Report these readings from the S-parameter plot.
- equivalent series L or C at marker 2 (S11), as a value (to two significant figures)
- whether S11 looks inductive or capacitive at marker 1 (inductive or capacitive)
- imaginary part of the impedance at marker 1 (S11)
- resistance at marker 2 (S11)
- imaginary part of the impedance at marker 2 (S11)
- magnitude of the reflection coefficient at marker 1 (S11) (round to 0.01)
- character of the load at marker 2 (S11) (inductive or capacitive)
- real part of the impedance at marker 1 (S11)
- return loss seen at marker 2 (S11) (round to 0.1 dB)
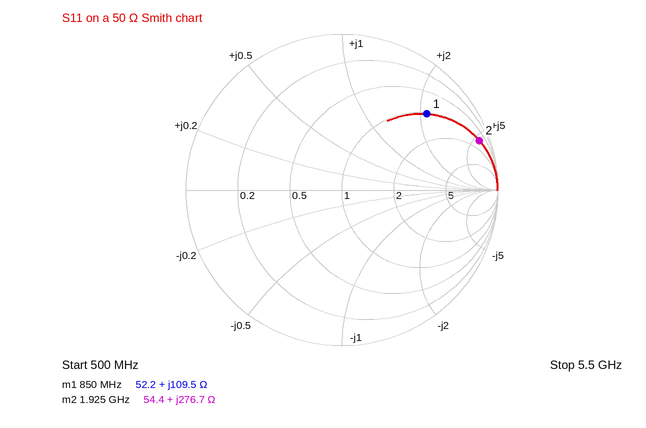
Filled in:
23 nH
inductive
+109.5 Ω
54.4 Ω
+276.7 Ω
0.73
inductive
52.2 Ω
0.6 dB
